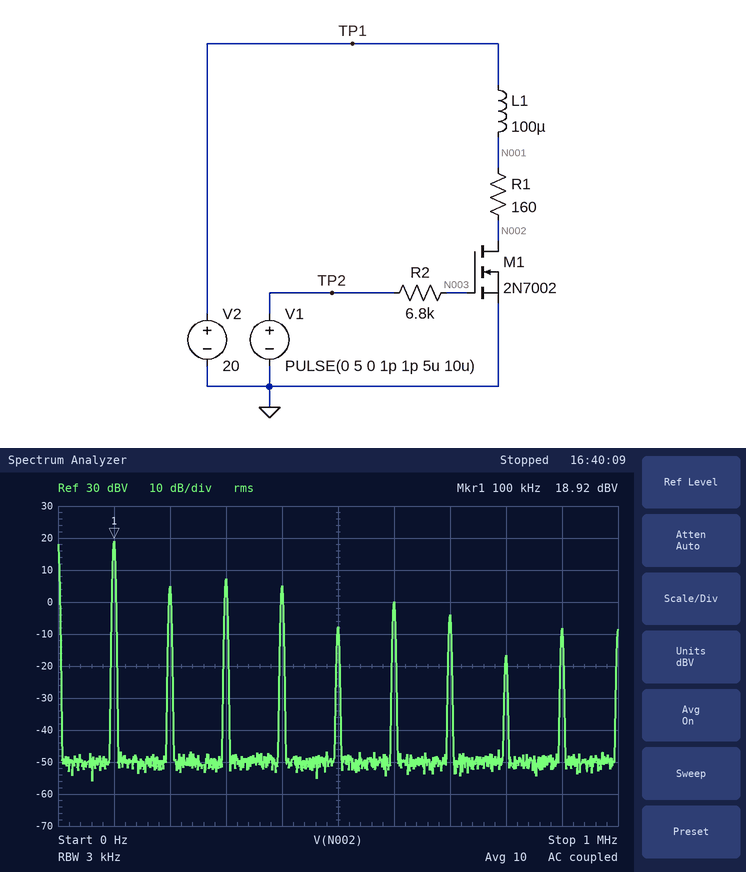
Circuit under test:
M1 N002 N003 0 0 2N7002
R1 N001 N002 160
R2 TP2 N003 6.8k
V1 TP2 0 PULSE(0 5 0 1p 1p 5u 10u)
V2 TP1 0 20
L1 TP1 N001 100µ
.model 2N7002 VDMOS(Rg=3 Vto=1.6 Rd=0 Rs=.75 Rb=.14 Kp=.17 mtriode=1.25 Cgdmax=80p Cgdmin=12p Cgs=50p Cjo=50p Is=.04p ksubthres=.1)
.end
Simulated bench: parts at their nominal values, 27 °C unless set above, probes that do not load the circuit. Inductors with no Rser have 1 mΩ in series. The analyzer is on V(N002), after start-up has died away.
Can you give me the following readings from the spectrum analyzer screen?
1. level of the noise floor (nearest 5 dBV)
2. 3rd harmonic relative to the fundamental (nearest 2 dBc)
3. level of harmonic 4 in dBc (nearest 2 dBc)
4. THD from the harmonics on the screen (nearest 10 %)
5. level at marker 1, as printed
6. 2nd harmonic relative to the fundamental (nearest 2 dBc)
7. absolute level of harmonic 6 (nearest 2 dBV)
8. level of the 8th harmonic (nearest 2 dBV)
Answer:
-50 dBV
-12 dBc
-14 dBc
40 %
18.92 dBV
-14 dBc
0 dBV
-16 dBV
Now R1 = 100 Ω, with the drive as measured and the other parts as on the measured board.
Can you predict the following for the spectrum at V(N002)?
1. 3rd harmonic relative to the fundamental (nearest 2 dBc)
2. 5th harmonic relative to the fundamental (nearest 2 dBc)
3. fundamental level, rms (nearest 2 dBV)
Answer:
-10 dBc
-20 dBc
20 dBV
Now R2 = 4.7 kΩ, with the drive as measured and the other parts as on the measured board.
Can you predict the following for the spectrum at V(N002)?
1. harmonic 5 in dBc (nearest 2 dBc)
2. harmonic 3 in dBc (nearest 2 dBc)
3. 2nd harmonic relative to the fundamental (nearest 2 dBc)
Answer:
-16 dBc
-10 dBc
-18 dBc
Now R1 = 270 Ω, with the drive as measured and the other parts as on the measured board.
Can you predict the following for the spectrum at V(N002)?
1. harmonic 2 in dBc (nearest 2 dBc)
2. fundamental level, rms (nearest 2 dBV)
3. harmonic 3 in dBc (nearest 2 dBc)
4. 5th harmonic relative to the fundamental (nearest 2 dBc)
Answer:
-12 dBc
18 dBV
-14 dBc
-38 dBc
